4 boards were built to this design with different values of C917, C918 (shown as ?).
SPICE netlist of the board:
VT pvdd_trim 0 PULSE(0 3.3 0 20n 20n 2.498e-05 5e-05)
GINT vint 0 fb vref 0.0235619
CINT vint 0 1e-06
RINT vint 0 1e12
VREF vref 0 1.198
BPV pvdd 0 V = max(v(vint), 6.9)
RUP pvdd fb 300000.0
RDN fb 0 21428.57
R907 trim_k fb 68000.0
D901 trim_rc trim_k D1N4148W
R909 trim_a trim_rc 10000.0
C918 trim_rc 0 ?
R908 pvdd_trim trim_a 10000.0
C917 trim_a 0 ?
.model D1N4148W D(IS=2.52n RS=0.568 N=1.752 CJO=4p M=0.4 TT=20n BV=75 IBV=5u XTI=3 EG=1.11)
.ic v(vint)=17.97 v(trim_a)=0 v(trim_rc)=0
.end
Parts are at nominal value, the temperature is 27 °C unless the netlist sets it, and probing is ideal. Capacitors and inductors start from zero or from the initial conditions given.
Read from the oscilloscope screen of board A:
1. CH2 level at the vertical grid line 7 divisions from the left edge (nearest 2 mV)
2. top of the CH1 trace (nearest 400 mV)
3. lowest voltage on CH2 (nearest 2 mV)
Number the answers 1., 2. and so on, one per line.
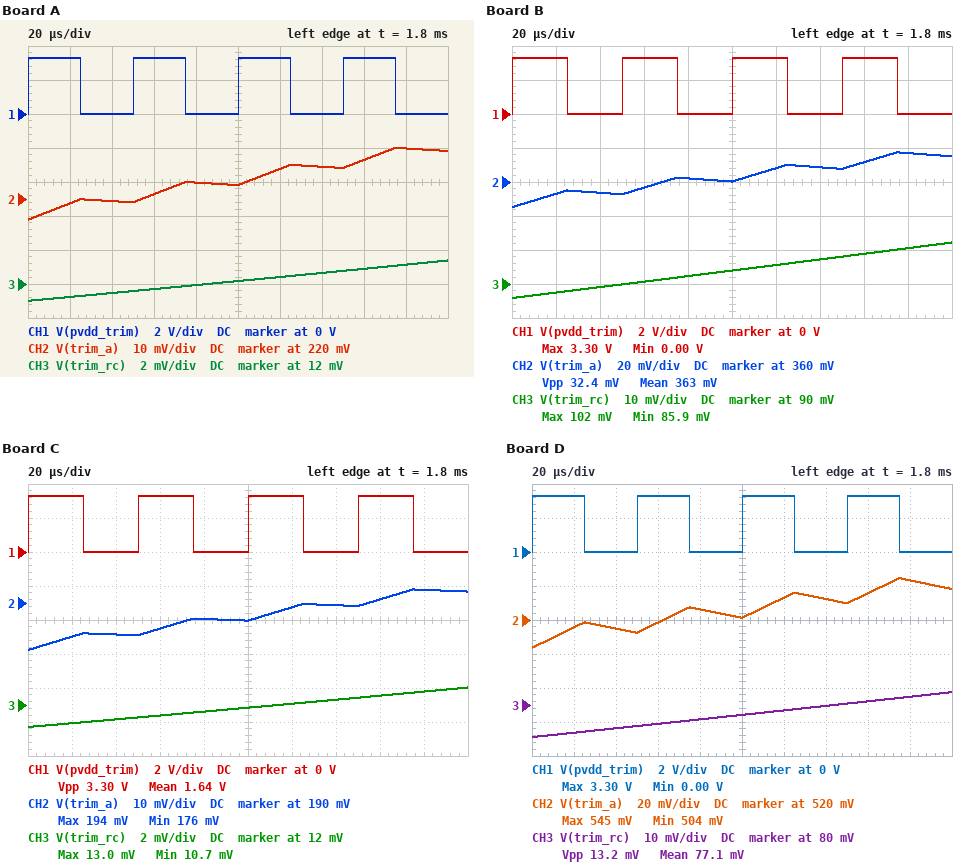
1. 230 mV
2. 3.2 V
3. 214 mV
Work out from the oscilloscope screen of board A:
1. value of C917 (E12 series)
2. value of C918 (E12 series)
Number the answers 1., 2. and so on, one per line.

1. 1.2 µF
2. 1.8 µF
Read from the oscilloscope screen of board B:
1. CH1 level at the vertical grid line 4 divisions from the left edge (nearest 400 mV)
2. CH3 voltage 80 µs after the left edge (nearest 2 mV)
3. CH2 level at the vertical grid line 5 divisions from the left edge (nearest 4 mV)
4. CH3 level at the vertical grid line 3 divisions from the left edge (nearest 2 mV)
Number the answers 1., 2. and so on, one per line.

1. 0 V
2. 92 mV
3. 360 mV
4. 90 mV
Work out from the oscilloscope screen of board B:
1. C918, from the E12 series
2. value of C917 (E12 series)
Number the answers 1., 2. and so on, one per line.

1. 330 nF
2. 680 nF
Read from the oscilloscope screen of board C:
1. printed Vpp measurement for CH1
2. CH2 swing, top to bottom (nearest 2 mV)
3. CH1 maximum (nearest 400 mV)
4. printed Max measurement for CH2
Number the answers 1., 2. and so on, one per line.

1. 3.30 V
2. 18 mV
3. 3.2 V
4. 194 mV
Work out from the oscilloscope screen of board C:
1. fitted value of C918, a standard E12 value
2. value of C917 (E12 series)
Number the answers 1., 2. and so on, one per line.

1. 1.5 µF
2. 1.5 µF
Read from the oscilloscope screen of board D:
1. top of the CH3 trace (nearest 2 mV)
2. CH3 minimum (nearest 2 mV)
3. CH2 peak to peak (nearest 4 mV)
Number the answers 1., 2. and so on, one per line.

1. 84 mV
2. 70 mV
3. 40 mV
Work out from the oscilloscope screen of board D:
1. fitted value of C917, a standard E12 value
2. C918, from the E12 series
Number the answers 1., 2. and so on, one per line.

1. 390 nF
2. 680 nF
